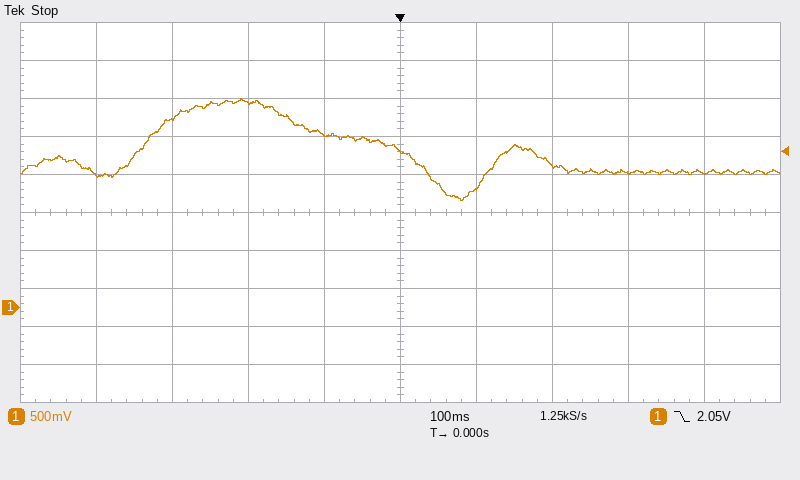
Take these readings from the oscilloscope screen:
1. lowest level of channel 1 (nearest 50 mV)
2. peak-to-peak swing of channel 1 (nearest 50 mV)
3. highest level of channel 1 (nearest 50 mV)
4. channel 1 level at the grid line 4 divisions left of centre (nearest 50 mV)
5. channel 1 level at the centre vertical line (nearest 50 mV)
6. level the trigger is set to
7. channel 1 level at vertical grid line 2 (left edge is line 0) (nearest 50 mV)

1.40 V
1.35 V
2.75 V
1.75 V
2.05 V
2.05 V
2.50 V
